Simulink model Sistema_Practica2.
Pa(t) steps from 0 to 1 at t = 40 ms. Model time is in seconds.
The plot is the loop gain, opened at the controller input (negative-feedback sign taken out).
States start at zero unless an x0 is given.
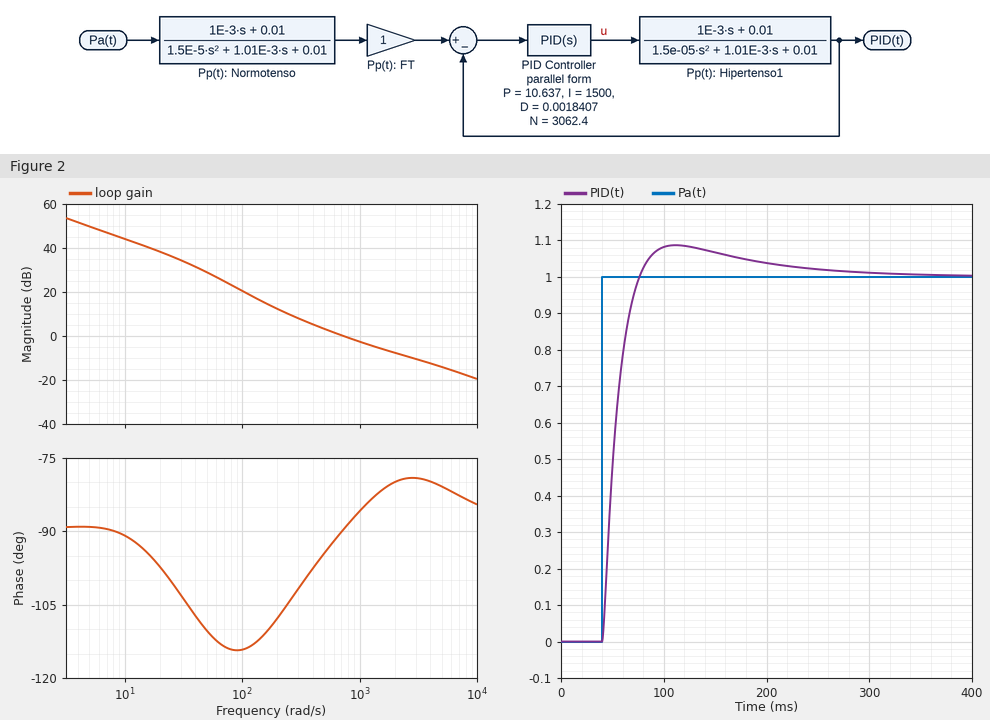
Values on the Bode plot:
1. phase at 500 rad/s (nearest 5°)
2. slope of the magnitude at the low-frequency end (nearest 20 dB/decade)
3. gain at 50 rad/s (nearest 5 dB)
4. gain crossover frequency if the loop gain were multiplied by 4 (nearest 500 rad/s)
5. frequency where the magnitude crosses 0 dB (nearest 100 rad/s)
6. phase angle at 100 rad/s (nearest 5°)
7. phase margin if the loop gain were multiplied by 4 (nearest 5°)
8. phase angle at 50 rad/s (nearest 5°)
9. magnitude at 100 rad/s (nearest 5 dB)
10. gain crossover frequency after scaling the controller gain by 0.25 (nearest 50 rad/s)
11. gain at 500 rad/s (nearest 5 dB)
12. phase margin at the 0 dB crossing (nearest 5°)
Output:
-95°
-20 dB/decade
30 dB
4000 rad/s
700 rad/s
-115°
100°
-110°
20 dB
200 rad/s
5 dB
90°
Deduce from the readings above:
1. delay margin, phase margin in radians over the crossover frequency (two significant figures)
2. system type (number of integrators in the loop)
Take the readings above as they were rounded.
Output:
0.0022 s
1
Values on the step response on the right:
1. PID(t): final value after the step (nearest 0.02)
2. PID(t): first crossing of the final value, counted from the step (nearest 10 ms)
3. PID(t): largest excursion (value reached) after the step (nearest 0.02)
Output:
1.00
40 ms
1.08
